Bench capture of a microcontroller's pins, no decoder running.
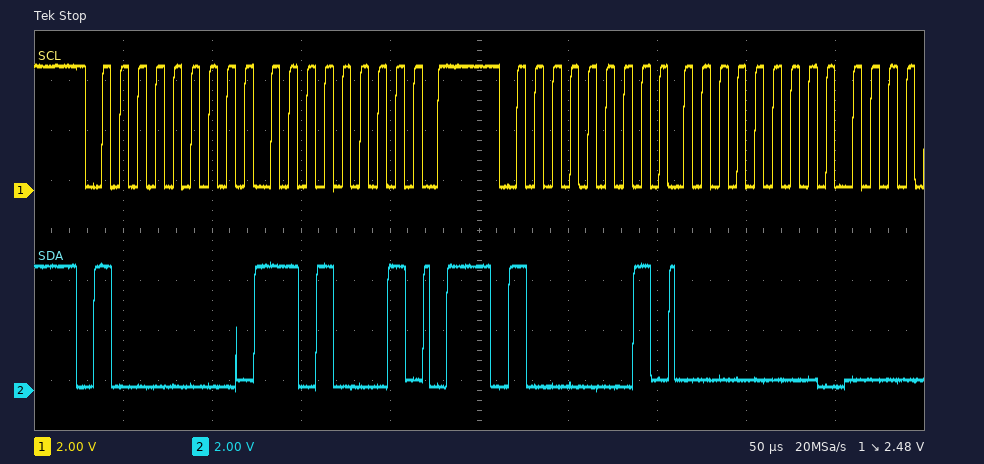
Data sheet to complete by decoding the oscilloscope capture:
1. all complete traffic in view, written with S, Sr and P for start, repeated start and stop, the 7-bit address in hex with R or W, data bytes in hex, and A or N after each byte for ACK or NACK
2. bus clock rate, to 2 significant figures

S 40W A D1 A P S 40R A 00 A
100 kHz
